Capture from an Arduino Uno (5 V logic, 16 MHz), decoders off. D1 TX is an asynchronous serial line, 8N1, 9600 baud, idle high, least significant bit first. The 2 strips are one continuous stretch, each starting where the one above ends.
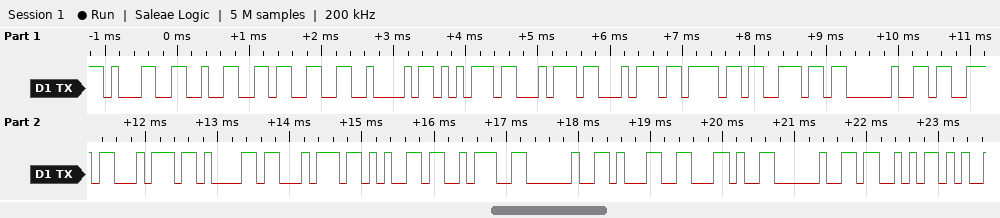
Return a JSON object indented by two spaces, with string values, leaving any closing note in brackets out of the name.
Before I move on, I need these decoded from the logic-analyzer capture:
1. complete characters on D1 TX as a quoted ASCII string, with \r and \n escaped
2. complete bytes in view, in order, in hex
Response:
{
  "complete characters on D1 TX as a quoted ASCII string, with \\r and \\n escaped": "\"123Button state: 1, S\"",
  "complete bytes in view, in order, in hex": "31 32 33 42 75 74 74 6F 6E 20 73 74 61 74 65 3A 20 31 2C 20 53"
}
